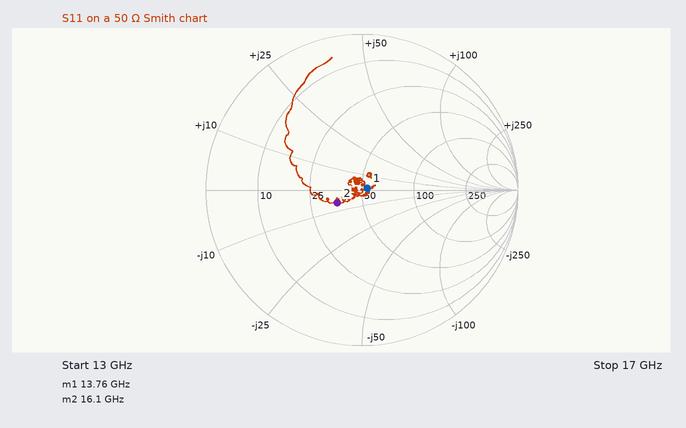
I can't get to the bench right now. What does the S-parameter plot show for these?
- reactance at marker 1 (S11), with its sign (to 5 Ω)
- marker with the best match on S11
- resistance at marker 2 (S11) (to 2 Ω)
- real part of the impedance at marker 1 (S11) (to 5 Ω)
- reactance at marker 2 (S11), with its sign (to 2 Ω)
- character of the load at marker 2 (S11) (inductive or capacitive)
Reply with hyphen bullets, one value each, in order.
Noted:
- 0 Ω
- marker 1
- 36 Ω
- 55 Ω
- -6 Ω
- capacitive
